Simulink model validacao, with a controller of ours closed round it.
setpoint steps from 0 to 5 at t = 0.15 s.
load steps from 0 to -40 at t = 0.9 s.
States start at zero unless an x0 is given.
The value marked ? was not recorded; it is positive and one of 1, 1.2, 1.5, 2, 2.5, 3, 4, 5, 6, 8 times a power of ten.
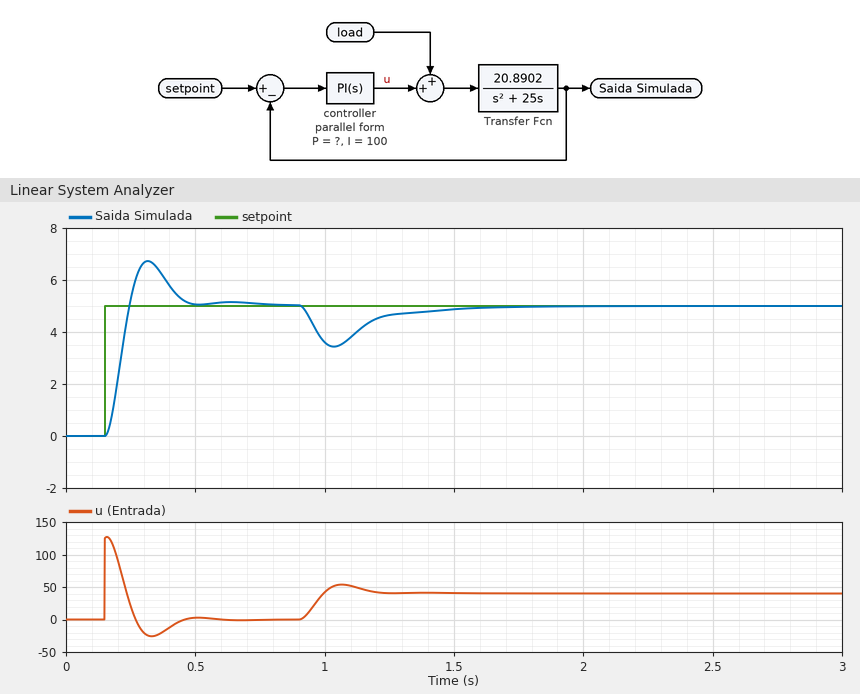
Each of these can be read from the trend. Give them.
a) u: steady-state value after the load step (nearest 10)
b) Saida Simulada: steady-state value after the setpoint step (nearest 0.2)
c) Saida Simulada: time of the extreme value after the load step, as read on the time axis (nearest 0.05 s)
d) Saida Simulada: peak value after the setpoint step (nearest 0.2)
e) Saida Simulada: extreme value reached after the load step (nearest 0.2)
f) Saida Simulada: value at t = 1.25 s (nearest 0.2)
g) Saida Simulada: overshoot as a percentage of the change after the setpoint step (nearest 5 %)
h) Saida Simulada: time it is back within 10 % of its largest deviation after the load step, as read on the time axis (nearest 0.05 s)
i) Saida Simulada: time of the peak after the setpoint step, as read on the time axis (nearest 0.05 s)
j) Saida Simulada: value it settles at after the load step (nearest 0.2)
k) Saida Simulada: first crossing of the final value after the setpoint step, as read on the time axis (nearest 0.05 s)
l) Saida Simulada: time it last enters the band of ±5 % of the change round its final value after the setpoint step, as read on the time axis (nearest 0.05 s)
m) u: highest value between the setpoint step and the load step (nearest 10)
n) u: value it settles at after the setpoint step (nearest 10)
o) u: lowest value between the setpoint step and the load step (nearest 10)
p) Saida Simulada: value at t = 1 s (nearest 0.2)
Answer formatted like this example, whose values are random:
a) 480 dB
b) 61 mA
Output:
a) 40
b) 5.0
c) 1.05 s
d) 6.8
e) 3.4
f) 4.6
g) 35 %
h) 1.45 s
i) 0.30 s
j) 5.0
k) 0.25 s
l) 0.45 s
m) 130
n) 0
o) -30
p) 3.6
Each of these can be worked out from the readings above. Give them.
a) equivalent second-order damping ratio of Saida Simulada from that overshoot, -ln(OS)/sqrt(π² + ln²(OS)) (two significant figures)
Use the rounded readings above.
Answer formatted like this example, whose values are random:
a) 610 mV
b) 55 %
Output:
a) 0.32
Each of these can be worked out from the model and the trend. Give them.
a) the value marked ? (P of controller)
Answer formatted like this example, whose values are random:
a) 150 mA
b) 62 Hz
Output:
a) 25
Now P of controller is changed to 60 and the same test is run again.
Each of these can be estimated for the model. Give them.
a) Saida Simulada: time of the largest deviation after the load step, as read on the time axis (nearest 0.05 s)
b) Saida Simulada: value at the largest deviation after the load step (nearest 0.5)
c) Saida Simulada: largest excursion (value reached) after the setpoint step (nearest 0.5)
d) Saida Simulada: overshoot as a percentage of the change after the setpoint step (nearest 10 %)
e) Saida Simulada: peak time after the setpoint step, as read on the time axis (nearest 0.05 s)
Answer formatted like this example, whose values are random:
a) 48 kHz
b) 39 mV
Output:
a) 1.00 s
b) 4.0
c) 7.0
d) 40 %
e) 0.25 s
